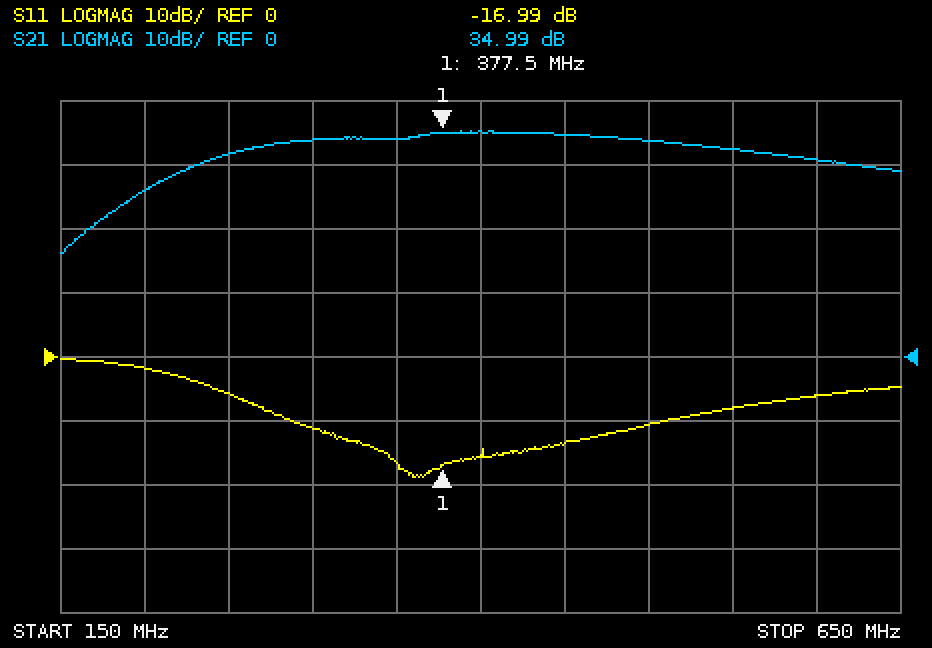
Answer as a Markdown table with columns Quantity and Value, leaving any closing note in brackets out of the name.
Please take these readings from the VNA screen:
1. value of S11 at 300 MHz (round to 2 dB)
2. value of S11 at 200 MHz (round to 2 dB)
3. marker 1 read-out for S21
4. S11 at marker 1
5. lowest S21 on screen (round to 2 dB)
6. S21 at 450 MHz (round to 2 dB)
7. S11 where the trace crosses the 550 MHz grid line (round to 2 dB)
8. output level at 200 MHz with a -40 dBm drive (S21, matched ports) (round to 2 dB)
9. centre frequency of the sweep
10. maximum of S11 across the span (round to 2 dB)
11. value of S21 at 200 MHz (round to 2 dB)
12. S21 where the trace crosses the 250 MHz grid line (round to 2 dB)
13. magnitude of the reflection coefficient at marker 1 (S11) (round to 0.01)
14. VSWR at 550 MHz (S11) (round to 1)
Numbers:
| Quantity | Value |
|---|---|
| value of S11 at 300 MHz | -12 dB |
| value of S11 at 200 MHz | -2 dB |
| marker 1 read-out for S21 | 34.99 dB |
| S11 at marker 1 | -16.99 dB |
| lowest S21 on screen | 16 dB |
| S21 at 450 MHz | 34 dB |
| S11 where the trace crosses the 550 MHz grid line | -8 dB |
| output level at 200 MHz with a -40 dBm drive (S21, matched ports) | -14 dBm |
| centre frequency of the sweep | 400 MHz |
| maximum of S11 across the span | 0 dB |
| value of S21 at 200 MHz | 26 dB |
| S21 where the trace crosses the 250 MHz grid line | 32 dB |
| magnitude of the reflection coefficient at marker 1 (S11) | 0.14 |
| VSWR at 550 MHz (S11) | 2 |
